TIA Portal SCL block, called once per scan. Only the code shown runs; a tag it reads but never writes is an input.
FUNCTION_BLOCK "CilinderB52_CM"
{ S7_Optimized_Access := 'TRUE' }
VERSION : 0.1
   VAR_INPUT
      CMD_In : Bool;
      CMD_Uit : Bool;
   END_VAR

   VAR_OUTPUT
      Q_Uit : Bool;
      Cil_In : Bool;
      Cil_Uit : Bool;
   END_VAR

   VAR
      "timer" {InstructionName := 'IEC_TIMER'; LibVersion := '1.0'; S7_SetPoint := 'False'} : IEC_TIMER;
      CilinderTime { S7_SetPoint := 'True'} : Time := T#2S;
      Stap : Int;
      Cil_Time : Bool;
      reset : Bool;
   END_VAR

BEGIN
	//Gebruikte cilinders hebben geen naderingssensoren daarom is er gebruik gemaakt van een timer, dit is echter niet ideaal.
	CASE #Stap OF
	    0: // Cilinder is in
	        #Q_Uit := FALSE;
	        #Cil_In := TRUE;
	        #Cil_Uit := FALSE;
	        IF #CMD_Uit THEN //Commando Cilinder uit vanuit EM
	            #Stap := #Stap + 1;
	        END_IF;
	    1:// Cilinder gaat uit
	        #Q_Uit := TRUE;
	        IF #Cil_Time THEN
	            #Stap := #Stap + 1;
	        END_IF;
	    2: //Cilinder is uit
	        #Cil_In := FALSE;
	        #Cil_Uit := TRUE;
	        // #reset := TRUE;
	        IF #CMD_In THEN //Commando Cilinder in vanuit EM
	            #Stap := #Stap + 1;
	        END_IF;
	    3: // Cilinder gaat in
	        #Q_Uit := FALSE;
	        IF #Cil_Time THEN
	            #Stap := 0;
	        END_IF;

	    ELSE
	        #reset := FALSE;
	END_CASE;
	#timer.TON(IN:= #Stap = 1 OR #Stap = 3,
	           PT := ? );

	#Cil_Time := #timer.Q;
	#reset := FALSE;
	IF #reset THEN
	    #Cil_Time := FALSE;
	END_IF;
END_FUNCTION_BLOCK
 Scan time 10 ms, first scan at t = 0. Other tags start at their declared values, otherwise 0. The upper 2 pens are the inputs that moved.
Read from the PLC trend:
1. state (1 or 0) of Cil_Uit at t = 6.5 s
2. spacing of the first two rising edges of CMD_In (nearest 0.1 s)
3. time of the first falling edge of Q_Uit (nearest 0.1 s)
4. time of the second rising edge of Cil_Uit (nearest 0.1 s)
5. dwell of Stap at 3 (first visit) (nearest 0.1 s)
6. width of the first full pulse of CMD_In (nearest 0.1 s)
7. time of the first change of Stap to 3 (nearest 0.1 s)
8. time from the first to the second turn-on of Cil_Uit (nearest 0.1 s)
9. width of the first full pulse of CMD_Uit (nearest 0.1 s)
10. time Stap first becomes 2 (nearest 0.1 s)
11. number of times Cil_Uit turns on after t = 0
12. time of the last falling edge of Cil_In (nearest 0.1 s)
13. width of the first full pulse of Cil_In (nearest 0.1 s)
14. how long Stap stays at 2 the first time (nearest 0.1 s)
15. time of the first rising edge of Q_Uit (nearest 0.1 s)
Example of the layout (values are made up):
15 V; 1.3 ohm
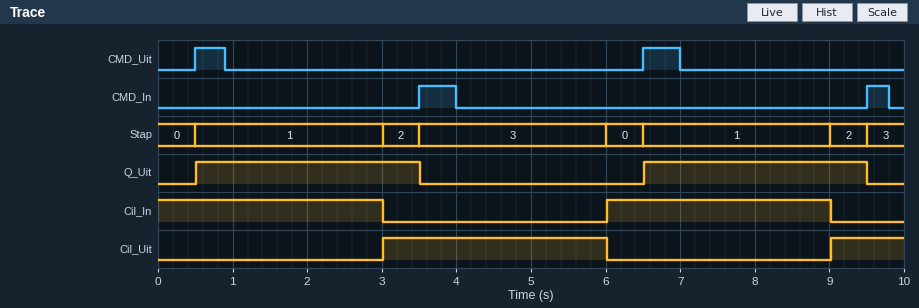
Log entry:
0; 6.0 s; 3.5 s; 9.0 s; 2.5 s; 0.5 s; 3.5 s; 6.0 s; 0.4 s; 3.0 s; 2; 9.0 s; 3.0 s; 0.5 s; 0.5 s
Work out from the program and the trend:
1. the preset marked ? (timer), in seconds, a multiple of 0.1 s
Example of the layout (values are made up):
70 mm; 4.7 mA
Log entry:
2.5 s
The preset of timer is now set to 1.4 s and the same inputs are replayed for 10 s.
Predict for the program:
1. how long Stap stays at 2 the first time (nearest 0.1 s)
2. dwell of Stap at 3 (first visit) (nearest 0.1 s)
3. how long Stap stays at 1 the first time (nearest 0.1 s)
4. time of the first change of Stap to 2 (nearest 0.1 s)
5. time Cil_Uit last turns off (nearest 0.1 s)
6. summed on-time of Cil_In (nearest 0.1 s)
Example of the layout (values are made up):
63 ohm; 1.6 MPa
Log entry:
1.6 s; 1.4 s; 1.4 s; 1.9 s; 4.9 s; 4.9 s
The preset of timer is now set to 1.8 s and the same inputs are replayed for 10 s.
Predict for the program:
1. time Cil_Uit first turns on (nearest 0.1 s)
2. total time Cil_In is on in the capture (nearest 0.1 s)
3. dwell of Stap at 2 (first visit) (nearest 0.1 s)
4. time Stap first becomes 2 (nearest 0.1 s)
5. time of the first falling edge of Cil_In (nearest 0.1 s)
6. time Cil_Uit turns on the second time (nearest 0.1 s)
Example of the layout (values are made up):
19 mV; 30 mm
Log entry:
2.3 s; 5.3 s; 1.2 s; 2.3 s; 2.3 s; 8.3 s
